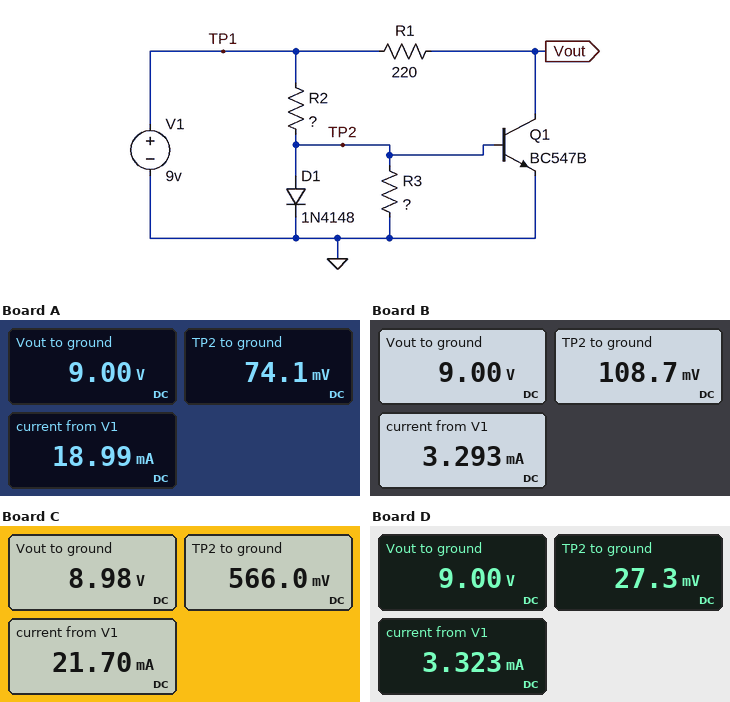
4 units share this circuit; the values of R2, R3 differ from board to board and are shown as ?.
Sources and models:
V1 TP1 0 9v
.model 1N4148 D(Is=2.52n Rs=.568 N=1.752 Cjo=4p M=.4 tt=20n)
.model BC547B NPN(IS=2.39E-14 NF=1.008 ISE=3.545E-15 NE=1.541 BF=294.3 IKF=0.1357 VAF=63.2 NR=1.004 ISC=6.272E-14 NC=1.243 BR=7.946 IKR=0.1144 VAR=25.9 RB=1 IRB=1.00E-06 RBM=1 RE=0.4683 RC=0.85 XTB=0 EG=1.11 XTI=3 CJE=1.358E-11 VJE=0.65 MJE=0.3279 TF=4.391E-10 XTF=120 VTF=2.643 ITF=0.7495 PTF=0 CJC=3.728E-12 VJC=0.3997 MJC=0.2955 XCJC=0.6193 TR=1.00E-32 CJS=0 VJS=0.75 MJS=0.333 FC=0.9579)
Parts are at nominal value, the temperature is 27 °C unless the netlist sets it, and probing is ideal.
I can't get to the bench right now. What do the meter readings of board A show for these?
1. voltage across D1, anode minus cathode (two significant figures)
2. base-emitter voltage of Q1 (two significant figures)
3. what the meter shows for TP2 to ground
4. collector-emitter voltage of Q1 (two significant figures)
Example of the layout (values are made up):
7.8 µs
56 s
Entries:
74 mV
74 mV
74.1 mV
9.0 V
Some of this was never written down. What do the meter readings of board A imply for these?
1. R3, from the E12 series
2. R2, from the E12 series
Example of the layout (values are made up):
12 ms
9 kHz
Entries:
3.9 Ω
470 Ω
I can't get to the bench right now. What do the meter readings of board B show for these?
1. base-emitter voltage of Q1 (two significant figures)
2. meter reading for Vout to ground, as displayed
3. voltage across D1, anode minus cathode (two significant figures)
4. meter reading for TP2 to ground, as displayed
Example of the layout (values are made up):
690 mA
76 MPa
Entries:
110 mV
9.00 V
110 mV
108.7 mV
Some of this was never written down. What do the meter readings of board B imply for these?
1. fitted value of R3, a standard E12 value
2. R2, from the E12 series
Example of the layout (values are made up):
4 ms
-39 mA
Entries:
33 Ω
2.7 kΩ
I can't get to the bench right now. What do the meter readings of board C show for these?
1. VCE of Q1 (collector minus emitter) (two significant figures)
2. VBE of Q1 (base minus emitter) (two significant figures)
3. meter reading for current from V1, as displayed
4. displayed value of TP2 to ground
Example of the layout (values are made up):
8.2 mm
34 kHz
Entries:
9.0 V
570 mV
21.70 mA
566.0 mV
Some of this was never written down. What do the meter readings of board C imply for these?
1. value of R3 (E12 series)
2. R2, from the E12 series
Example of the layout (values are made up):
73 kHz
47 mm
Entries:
27 Ω
390 Ω
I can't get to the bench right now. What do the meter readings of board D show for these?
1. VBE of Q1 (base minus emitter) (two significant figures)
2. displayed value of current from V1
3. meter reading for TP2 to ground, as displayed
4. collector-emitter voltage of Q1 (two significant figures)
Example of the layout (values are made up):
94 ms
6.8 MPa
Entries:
27 mV
3.323 mA
27.3 mV
9.0 V
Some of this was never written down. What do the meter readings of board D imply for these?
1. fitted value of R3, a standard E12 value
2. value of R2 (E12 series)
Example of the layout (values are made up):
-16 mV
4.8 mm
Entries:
8.2 Ω
2.7 kΩ
